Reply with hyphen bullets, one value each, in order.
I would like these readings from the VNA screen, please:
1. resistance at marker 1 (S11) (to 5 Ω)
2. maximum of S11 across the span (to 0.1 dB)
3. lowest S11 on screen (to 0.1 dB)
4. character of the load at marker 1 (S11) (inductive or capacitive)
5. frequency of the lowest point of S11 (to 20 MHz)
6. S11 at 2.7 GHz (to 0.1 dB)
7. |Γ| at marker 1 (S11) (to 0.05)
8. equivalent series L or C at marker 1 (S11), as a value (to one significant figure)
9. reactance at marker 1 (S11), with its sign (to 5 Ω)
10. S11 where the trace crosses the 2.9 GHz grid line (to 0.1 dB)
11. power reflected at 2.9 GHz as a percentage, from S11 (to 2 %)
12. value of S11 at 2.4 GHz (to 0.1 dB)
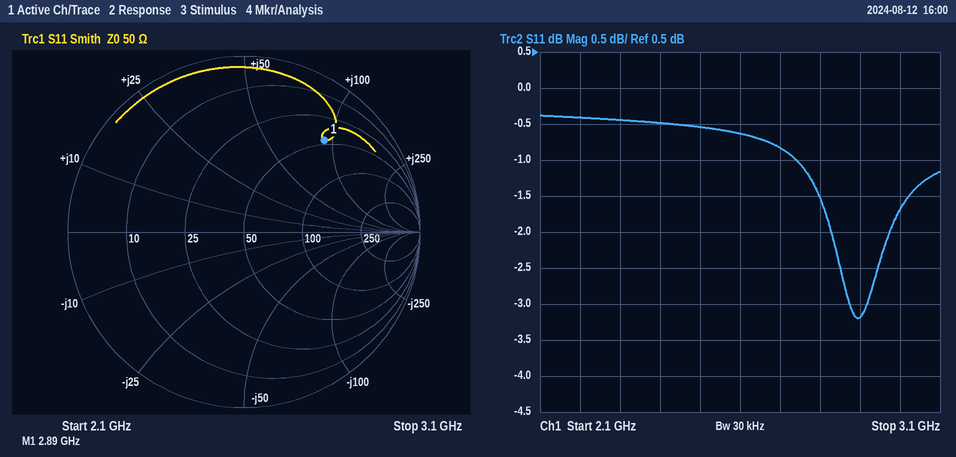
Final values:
- 45 Ω
- -0.4 dB
- -3.2 dB
- inductive
- 2.90 GHz
- -0.8 dB
- 0.70
- 5 nH
- +90 Ω
- -3.2 dB
- 48 %
- -0.5 dB
